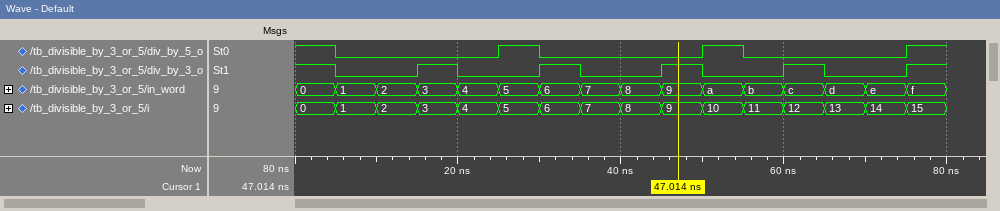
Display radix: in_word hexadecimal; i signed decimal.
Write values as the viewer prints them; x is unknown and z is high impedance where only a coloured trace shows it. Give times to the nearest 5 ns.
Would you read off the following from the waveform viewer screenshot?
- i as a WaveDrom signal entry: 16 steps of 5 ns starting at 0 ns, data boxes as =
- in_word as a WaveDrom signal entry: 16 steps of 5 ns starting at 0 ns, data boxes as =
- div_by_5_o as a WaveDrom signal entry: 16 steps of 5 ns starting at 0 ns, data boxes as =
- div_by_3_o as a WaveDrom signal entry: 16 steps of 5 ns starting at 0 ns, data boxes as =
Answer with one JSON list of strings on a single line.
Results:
["{name: 'i', wave: '================', data: '0 1 2 3 4 5 6 7 8 9 10 11 12 13 14 15'}", "{name: 'in_word', wave: '================', data: '0 1 2 3 4 5 6 7 8 9 a b c d e f'}", "{name: 'div_by_5_o', wave: '10...10...10...1'}", "{name: 'div_by_3_o', wave: '10.10.10.10.10.1'}"]
